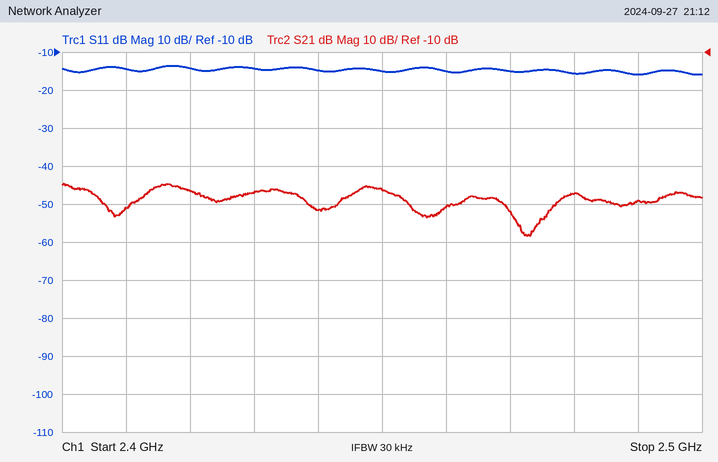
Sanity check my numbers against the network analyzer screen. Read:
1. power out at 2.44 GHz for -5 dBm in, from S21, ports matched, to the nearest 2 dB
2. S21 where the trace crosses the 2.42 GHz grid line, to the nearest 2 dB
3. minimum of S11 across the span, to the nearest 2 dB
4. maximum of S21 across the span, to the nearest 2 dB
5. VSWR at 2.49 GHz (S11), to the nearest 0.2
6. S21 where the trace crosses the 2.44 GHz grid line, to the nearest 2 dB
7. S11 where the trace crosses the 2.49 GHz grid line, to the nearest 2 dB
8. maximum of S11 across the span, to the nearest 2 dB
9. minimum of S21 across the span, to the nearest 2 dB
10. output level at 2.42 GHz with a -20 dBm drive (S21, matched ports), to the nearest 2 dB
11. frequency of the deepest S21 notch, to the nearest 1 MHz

-56 dBm
-46 dB
-16 dB
-44 dB
1.4
-52 dB
-16 dB
-14 dB
-58 dB
-66 dBm
2.473 GHz
